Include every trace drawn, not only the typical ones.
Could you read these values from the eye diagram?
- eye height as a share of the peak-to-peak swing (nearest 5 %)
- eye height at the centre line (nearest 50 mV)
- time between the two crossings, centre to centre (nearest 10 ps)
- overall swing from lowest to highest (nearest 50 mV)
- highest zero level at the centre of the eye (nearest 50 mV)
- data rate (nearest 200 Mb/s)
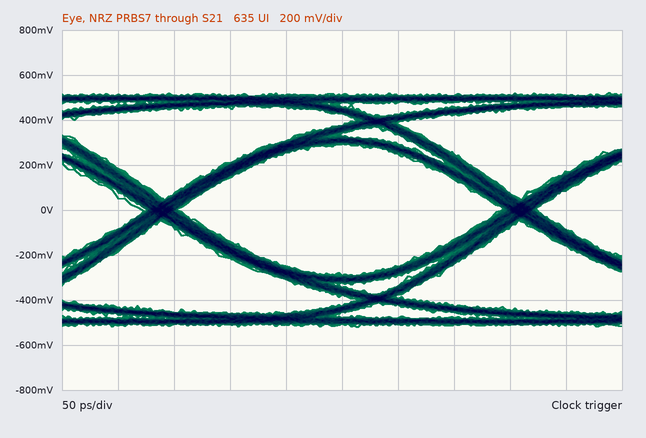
55 %
600 mV
320 ps
1.05 V
-300 mV
3.2 Gb/s
